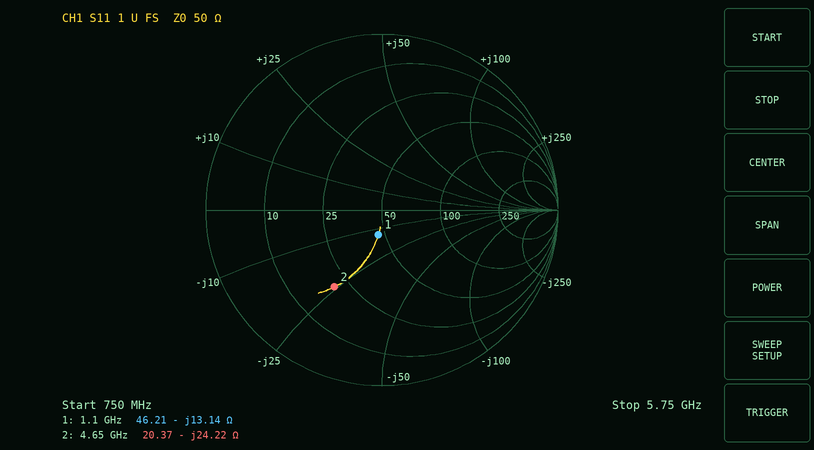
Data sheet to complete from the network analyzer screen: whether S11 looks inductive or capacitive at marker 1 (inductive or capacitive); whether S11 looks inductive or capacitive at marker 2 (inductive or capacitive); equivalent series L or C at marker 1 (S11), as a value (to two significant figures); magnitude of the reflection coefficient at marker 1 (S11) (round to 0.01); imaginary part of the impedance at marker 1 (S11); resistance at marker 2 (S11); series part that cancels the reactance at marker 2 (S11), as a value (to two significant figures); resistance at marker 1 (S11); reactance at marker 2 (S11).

capacitive
capacitive
11 pF
0.14
-13.14 Ω
20.37 Ω
830 pH
46.21 Ω
-24.22 Ω
